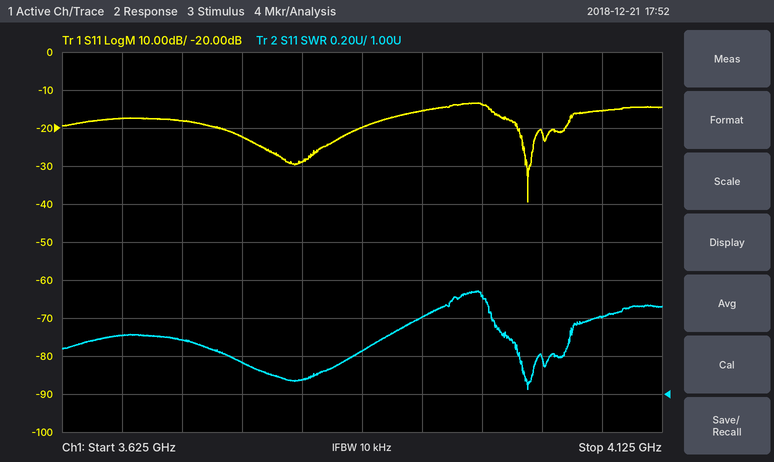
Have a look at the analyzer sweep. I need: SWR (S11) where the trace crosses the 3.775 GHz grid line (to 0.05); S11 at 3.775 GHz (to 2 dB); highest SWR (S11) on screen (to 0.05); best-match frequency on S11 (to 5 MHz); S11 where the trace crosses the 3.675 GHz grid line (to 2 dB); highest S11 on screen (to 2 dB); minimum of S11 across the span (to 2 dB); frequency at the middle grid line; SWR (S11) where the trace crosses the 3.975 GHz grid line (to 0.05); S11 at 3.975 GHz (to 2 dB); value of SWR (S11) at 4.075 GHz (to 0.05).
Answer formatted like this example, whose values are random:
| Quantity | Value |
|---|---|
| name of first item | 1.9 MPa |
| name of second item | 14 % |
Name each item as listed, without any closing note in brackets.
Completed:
| Quantity | Value |
|---|---|
| SWR (S11) where the trace crosses the 3.775 GHz grid line | 1.15 |
| S11 at 3.775 GHz | -22 dB |
| highest SWR (S11) on screen | 1.55 |
| best-match frequency on S11 | 4.015 GHz |
| S11 where the trace crosses the 3.675 GHz grid line | -18 dB |
| highest S11 on screen | -14 dB |
| minimum of S11 across the span | -40 dB |
| frequency at the middle grid line | 3.875 GHz |
| SWR (S11) where the trace crosses the 3.975 GHz grid line | 1.50 |
| S11 at 3.975 GHz | -14 dB |
| value of SWR (S11) at 4.075 GHz | 1.40 |
